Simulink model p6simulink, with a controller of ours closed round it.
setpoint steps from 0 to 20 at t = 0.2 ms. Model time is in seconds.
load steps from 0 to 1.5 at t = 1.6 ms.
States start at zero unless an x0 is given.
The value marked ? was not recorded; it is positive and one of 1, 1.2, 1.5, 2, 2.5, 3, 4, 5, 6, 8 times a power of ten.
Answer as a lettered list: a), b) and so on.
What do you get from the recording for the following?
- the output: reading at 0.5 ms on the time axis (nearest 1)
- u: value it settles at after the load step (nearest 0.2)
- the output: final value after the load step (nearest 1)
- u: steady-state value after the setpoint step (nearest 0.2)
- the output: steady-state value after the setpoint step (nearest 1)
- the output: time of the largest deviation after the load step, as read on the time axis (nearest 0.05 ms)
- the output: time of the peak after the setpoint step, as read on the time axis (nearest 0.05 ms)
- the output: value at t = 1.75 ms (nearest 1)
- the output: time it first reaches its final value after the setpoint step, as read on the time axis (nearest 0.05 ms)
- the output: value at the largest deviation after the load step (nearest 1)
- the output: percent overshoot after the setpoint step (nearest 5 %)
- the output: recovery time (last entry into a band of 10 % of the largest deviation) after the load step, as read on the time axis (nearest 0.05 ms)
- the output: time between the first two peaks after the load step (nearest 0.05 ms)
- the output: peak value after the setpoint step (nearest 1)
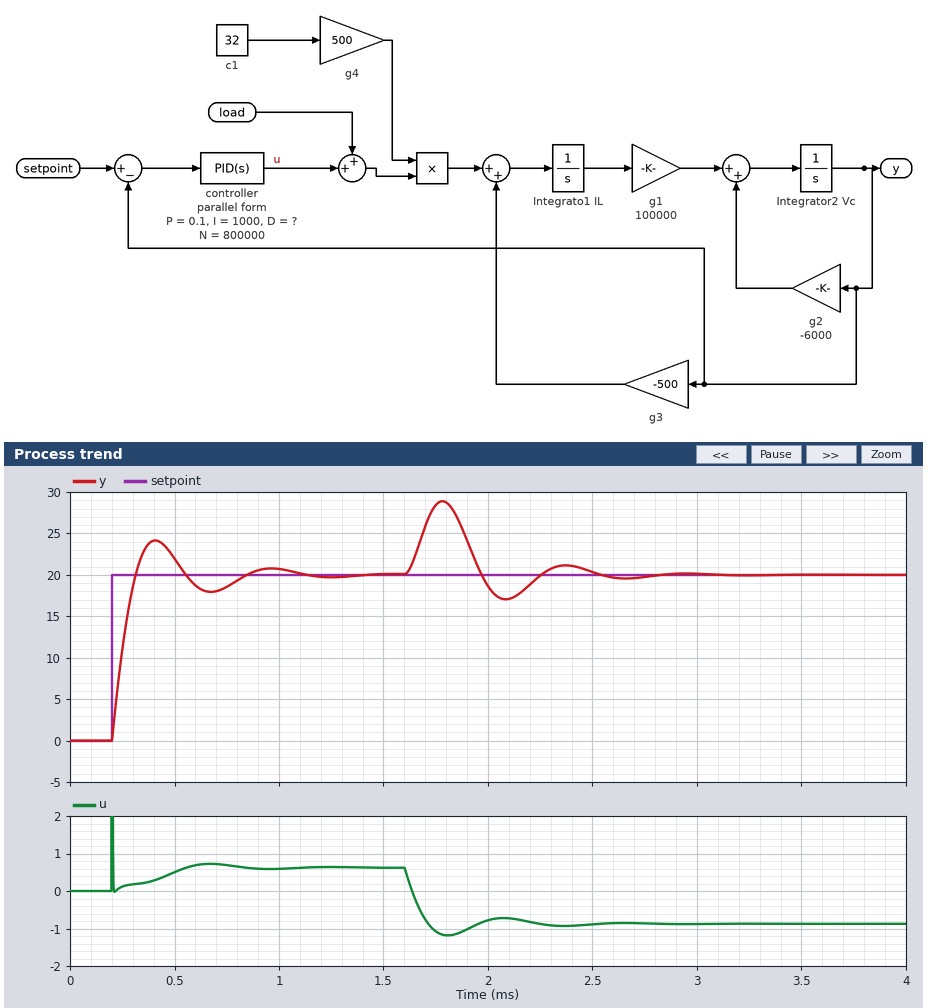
a) 22
b) -0.8
c) 20
d) 0.6
e) 20
f) 1.80 ms
g) 0.40 ms
h) 28
i) 0.30 ms
j) 29
k) 20 %
l) 2.45 ms
m) 0.60 ms
n) 24
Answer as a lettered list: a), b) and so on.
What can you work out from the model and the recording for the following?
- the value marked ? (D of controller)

a) 8e-06
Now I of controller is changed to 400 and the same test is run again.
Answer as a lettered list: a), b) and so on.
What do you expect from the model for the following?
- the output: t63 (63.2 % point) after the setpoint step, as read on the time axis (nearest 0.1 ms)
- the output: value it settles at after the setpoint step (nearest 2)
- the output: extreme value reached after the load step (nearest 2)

a) 0.3 ms
b) 20
c) 30
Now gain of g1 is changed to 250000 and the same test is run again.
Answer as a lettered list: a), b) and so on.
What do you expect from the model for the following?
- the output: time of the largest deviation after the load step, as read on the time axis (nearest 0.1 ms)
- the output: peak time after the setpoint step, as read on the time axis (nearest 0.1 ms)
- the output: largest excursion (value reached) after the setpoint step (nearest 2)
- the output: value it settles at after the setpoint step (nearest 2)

a) 1.7 ms
b) 0.3 ms
c) 20
d) 20
